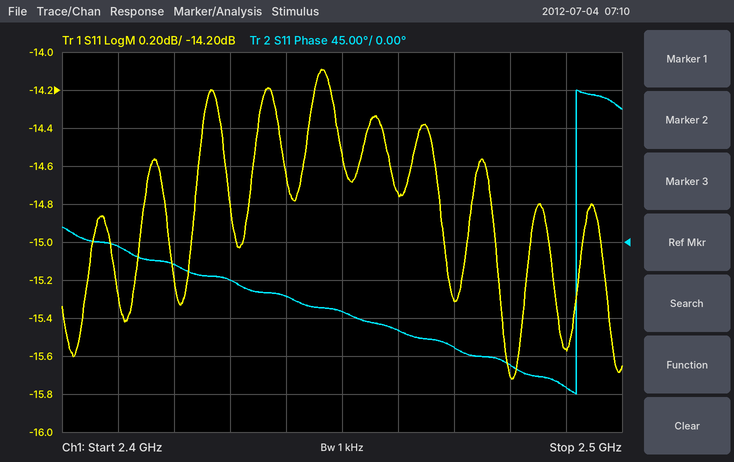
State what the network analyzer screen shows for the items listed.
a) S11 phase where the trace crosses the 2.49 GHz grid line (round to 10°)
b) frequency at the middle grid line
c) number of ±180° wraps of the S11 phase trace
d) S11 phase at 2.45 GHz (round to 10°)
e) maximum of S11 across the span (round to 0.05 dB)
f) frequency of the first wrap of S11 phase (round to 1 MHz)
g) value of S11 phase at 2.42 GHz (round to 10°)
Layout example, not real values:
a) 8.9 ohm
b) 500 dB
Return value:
a) -170°
b) 2.45 GHz
c) 1
d) -80°
e) -14.10 dB
f) 2.492 GHz
g) -30°
